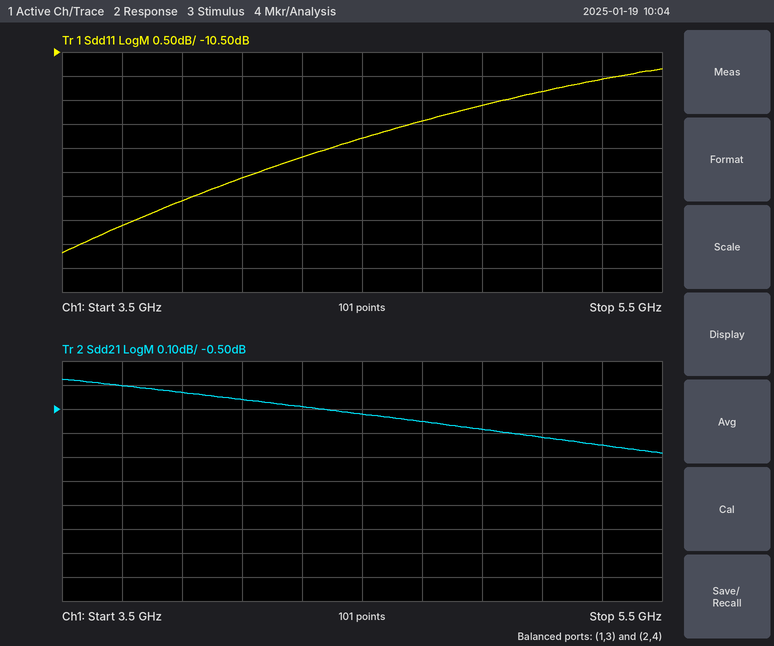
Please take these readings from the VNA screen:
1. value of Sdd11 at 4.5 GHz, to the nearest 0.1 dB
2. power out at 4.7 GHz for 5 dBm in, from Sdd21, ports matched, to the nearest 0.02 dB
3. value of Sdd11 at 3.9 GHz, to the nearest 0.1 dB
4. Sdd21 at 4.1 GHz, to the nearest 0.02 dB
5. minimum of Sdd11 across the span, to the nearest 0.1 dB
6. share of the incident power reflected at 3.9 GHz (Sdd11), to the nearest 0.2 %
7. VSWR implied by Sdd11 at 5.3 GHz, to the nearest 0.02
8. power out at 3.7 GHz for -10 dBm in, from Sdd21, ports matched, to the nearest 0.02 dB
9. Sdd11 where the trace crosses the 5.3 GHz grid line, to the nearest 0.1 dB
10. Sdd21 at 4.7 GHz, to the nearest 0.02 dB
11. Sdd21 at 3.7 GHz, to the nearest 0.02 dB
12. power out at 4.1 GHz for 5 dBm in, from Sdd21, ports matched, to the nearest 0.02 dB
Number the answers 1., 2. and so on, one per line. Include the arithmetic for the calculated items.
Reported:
1. -12.3 dB
2. 5 dBm + (-0.56 dB) = 4.44 dBm
3. -13.6 dB
4. -0.46 dB
5. -14.7 dB
6. 10^(-13.6/10) ≈ 4.4 %
7. |Γ| = 10^(-11.1/20) = 0.2786; VSWR = (1 + 0.2786)/(1 − 0.2786) ≈ 1.77, so 1.78 to the nearest 0.02
8. -10 dBm + (-0.40 dB) = -10.40 dBm
9. -11.1 dB
10. -0.56 dB
11. -0.40 dB
12. 5 dBm + (-0.46 dB) = 4.54 dBm
